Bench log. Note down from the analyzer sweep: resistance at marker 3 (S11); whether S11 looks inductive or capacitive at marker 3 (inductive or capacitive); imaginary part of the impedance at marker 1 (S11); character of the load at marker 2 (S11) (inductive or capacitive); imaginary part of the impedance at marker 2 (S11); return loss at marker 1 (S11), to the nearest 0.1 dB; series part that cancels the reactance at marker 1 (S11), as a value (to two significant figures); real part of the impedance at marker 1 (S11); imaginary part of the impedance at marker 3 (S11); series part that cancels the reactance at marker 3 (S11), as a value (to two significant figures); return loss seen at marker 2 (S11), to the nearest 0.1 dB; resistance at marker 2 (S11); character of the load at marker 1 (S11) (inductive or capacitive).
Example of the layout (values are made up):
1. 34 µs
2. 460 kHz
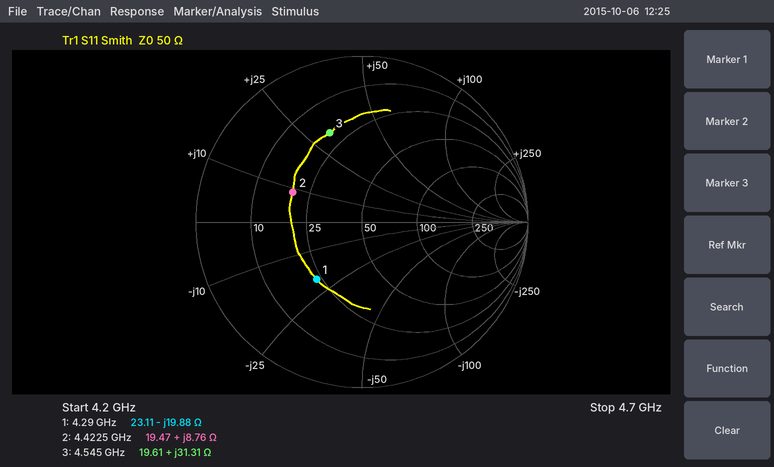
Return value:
1. 19.61 Ω
2. inductive
3. -19.88 Ω
4. inductive
5. +8.76 Ω
6. 7.1 dB
7. 740 pH
8. 23.11 Ω
9. +31.31 Ω
10. 1.1 pF
11. 6.9 dB
12. 19.47 Ω
13. capacitive
